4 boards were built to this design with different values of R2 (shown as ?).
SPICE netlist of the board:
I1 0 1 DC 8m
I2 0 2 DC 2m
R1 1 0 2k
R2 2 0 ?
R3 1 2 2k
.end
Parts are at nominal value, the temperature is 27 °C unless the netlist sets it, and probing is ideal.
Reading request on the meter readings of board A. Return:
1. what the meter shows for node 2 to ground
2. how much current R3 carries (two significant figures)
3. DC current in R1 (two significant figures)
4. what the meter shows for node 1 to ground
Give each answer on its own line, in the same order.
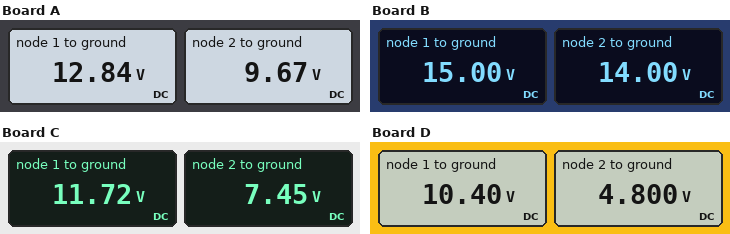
9.67 V
1.6 mA
6.4 mA
12.84 V
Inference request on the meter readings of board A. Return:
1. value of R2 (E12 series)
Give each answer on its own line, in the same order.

2.7 kΩ
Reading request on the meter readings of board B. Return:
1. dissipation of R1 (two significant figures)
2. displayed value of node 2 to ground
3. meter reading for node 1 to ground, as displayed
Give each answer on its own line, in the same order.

110 mW
14.00 V
15.00 V
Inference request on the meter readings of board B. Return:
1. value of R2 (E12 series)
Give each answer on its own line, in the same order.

5.6 kΩ
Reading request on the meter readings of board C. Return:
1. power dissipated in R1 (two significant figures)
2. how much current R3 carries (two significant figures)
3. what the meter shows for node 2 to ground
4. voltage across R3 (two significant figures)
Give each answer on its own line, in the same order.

69 mW
2.1 mA
7.45 V
4.3 V
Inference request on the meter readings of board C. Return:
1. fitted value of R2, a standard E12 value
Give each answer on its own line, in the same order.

1.8 kΩ
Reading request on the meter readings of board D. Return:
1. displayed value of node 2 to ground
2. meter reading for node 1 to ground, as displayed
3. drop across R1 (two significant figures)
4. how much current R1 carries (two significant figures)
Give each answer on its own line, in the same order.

4.800 V
10.40 V
10 V
5.2 mA
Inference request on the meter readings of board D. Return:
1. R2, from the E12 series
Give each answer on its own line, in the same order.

1 kΩ
